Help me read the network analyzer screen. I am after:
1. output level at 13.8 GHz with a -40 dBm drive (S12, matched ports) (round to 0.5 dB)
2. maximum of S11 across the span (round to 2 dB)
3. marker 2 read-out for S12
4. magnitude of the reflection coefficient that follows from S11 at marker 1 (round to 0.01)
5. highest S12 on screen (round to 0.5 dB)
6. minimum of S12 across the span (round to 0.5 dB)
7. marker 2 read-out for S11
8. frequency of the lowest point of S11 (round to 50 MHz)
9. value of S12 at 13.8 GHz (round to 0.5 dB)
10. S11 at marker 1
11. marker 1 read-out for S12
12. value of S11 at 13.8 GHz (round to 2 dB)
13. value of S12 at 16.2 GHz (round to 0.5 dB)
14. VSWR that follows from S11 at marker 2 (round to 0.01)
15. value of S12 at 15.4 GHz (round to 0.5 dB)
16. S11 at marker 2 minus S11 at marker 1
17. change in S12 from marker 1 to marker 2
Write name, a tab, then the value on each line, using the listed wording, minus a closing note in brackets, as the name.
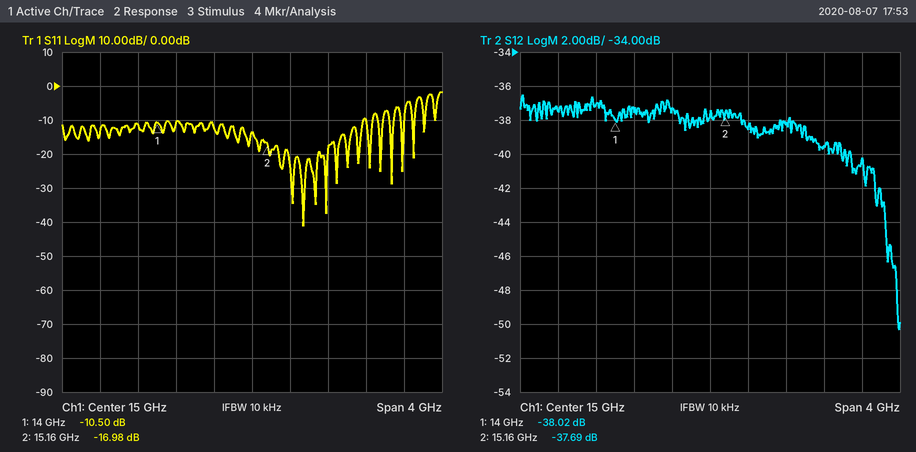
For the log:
output level at 13.8 GHz with a -40 dBm drive (S12, matched ports)	-77.0 dBm
maximum of S11 across the span	-2 dB
marker 2 read-out for S12	-37.69 dB
magnitude of the reflection coefficient that follows from S11 at marker 1	0.30
highest S12 on screen	-36.5 dB
minimum of S12 across the span	-50.5 dB
marker 2 read-out for S11	-16.98 dB
frequency of the lowest point of S11	15.55 GHz
value of S12 at 13.8 GHz	-37.0 dB
S11 at marker 1	-10.50 dB
marker 1 read-out for S12	-38.02 dB
value of S11 at 13.8 GHz	-12 dB
value of S12 at 16.2 GHz	-39.5 dB
VSWR that follows from S11 at marker 2	1.33
value of S12 at 15.4 GHz	-38.5 dB
S11 at marker 2 minus S11 at marker 1	-6.48 dB
change in S12 from marker 1 to marker 2	0.33 dB
